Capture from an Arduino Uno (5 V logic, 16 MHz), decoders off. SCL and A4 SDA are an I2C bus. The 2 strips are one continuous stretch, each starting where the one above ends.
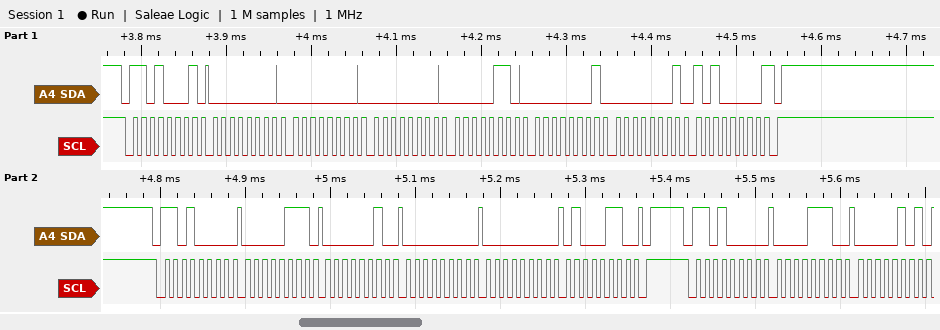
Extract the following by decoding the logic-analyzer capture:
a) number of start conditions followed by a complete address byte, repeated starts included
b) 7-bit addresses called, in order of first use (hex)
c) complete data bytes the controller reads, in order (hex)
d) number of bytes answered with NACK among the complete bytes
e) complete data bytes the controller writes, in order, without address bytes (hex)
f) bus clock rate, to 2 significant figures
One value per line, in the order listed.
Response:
3
0x68
00 00 00 06 01 01 A0
1
07 02 00 00 46 0E 05
100 kHz
